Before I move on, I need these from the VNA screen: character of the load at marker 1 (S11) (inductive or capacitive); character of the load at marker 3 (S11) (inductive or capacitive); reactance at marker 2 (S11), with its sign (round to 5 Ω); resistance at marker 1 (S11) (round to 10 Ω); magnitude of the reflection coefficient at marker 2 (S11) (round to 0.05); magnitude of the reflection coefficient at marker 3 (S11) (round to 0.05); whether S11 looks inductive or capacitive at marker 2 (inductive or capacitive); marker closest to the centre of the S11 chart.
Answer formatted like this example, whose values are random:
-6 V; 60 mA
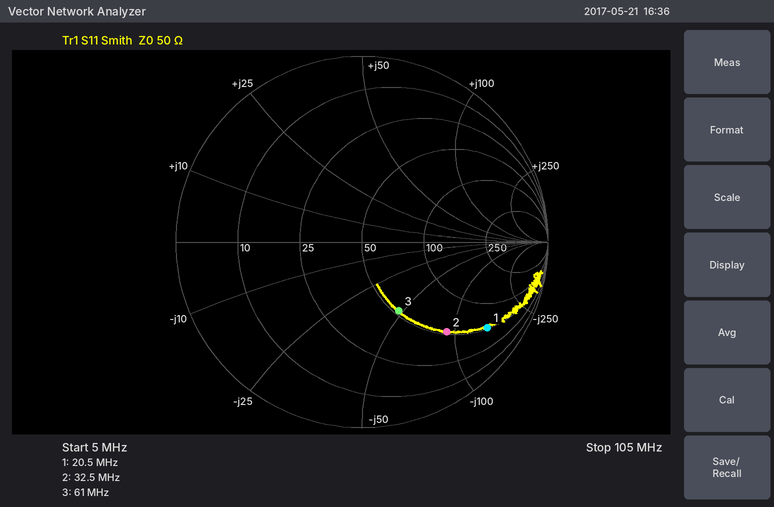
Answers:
capacitive; capacitive; -90 Ω; 50 Ω; 0.65; 0.40; capacitive; marker 3
